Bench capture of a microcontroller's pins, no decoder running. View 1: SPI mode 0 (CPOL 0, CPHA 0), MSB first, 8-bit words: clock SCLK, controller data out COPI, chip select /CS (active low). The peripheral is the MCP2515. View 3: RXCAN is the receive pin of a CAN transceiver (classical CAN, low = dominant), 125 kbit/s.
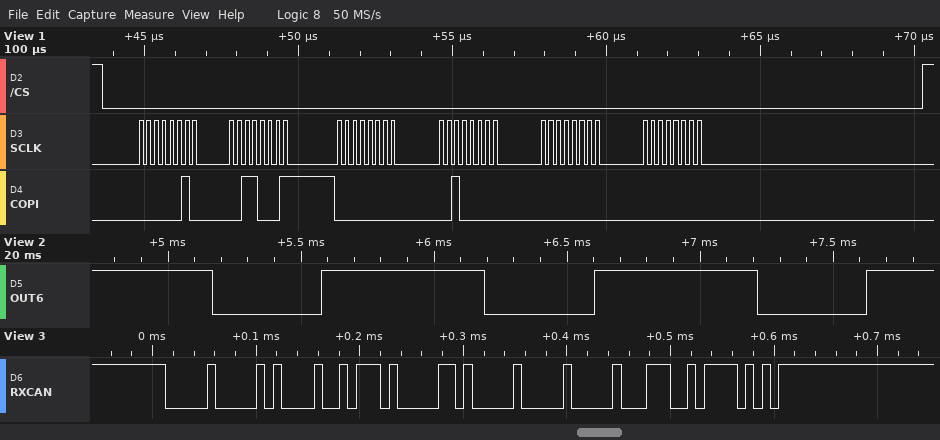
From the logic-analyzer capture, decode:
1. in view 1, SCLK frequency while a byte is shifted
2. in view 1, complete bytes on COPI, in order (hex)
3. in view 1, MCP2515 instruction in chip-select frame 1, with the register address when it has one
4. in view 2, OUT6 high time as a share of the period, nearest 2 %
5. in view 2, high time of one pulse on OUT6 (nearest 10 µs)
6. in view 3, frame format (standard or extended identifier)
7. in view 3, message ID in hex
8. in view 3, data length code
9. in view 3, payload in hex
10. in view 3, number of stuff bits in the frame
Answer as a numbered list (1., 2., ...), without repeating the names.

1. 4 MHz
2. 02 31 00 20 00 00
3. WRITE 0x31
4. 60 %
5. 610 µs
6. standard
7. 0x001
8. 4
9. BA 0A 00 00
10. 6
